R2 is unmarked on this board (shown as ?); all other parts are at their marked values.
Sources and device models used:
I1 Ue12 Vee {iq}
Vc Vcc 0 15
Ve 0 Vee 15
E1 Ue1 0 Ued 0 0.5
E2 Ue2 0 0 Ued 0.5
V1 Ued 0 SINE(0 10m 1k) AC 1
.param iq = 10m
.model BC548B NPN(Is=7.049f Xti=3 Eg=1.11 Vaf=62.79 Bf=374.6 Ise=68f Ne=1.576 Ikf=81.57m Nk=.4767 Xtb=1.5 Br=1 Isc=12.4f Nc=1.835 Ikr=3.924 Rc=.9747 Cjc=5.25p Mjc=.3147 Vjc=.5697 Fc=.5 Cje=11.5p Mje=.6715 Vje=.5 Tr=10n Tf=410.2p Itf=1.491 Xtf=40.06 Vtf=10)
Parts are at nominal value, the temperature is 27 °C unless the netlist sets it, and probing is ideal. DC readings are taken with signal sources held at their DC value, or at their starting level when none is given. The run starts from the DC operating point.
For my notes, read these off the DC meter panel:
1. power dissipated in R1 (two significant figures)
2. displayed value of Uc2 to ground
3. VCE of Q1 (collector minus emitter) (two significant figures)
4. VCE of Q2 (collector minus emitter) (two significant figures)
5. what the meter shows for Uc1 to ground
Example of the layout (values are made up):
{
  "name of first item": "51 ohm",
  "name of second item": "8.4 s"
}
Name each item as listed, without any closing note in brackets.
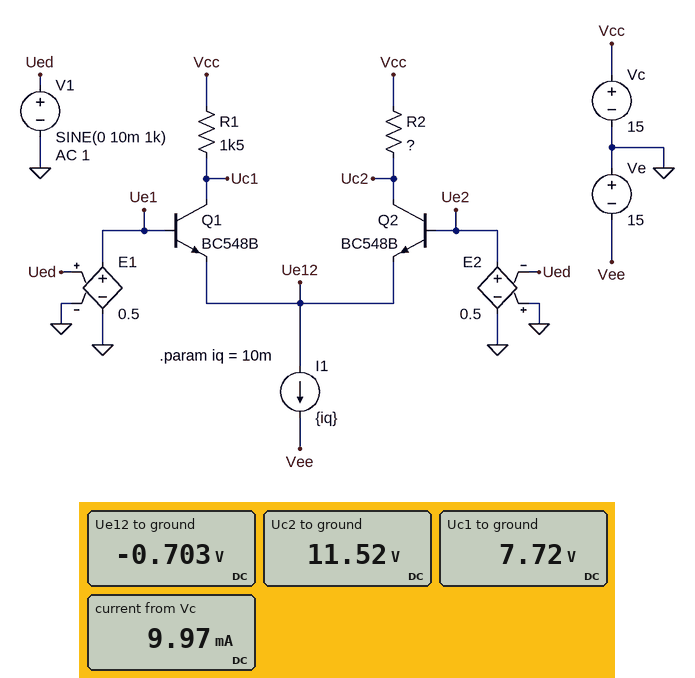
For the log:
{
  "power dissipated in R1": "35 mW",
  "displayed value of Uc2 to ground": "11.52 V",
  "VCE of Q1 (collector minus emitter)": "8.4 V",
  "VCE of Q2 (collector minus emitter)": "12 V",
  "what the meter shows for Uc1 to ground": "7.72 V"
}
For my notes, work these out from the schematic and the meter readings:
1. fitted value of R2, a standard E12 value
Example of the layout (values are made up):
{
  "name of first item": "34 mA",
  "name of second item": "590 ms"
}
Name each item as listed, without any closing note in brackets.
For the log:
{
  "fitted value of R2, a standard E12 value": "680 Ω"
}
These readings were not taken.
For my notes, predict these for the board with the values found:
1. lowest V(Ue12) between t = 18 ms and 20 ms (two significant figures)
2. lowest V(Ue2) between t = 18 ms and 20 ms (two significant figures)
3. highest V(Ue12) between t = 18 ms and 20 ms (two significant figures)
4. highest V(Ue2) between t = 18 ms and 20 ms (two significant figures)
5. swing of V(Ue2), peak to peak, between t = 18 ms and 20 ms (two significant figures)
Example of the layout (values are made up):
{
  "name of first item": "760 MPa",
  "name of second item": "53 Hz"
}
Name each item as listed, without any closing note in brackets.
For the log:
{
  "lowest V(Ue12) between t = 18 ms and 20 ms": "-700 mV",
  "lowest V(Ue2) between t = 18 ms and 20 ms": "-5.0 mV",
  "highest V(Ue12) between t = 18 ms and 20 ms": "-700 mV",
  "highest V(Ue2) between t = 18 ms and 20 ms": "5.0 mV",
  "swing of V(Ue2), peak to peak, between t = 18 ms and 20 ms": "10 mV"
}
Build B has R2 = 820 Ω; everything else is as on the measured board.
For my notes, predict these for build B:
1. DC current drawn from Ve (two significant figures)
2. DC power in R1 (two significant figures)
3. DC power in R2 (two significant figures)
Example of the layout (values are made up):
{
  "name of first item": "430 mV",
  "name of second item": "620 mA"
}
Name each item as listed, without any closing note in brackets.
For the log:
{
  "DC current drawn from Ve": "10 mA",
  "DC power in R1": "36 mW",
  "DC power in R2": "21 mW"
}
